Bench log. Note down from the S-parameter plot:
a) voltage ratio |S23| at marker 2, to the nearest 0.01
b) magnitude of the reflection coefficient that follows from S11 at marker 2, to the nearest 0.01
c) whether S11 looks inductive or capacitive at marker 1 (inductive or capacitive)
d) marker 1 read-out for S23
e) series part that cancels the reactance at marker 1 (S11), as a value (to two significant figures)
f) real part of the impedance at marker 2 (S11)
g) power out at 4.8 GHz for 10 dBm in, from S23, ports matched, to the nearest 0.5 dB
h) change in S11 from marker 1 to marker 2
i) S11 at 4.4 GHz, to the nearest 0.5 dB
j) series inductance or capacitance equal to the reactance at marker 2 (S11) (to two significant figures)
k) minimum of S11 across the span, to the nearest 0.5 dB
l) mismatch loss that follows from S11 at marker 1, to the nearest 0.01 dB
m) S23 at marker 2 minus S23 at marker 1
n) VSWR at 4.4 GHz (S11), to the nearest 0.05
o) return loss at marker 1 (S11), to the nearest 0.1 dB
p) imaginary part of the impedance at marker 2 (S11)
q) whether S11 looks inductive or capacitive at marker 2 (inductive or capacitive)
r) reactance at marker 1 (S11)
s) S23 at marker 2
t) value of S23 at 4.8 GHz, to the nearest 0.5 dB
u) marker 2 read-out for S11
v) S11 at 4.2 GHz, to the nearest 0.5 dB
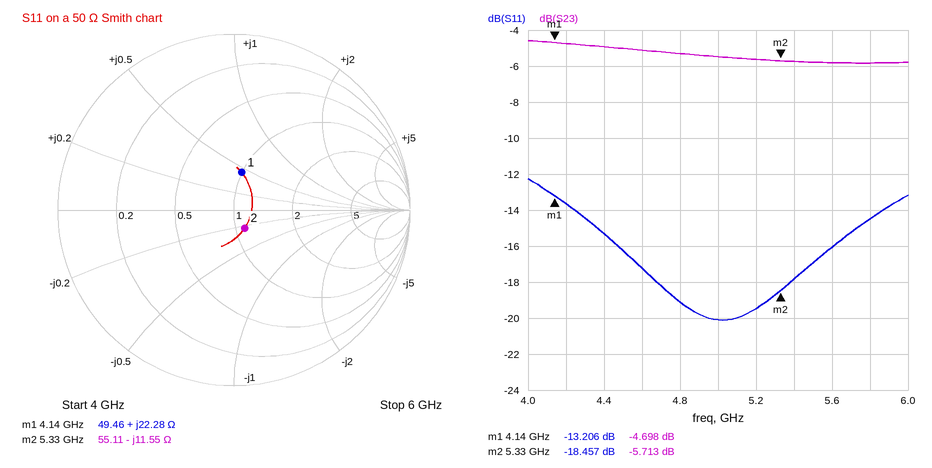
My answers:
0.52
0.12
inductive
-4.698 dB
1.7 pF
55.11 Ω
4.5 dBm
-5.251 dB
-15.5 dB
2.6 pF
-20.0 dB
0.21 dB
-1.015 dB
1.40
13.2 dB
-11.55 Ω
capacitive
+22.28 Ω
-5.713 dB
-5.5 dB
-18.457 dB
-13.5 dB
